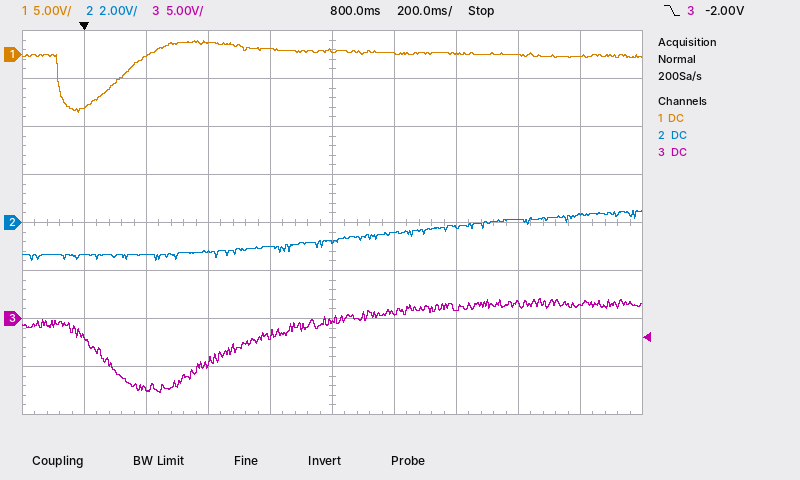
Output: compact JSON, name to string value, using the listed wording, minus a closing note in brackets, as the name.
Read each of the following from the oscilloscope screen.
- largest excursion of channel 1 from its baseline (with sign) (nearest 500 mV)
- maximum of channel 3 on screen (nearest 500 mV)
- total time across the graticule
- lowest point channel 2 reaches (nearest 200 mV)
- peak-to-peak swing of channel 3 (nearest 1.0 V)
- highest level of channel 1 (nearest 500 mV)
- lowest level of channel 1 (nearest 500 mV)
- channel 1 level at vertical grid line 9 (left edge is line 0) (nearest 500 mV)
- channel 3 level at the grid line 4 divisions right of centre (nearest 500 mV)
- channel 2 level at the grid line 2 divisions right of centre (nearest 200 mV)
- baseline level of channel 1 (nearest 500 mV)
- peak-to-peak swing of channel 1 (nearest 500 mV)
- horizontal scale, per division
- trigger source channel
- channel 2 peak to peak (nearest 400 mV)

{"largest excursion of channel 1 from its baseline (with sign)": "-6.0 V", "maximum of channel 3 on screen": "2.0 V", "total time across the graticule": "2 s", "lowest point channel 2 reaches": "-1.6 V", "peak-to-peak swing of channel 3": "10.0 V", "highest level of channel 1": "1.5 V", "lowest level of channel 1": "-6.0 V", "channel 1 level at vertical grid line 9 (left edge is line 0)": "0.0 V", "channel 3 level at the grid line 4 divisions right of centre": "1.5 V", "channel 2 level at the grid line 2 divisions right of centre": "-200 mV", "baseline level of channel 1": "0.0 V", "peak-to-peak swing of channel 1": "7.5 V", "horizontal scale, per division": "200 ms", "trigger source channel": "channel 3", "channel 2 peak to peak": "2.0 V"}
